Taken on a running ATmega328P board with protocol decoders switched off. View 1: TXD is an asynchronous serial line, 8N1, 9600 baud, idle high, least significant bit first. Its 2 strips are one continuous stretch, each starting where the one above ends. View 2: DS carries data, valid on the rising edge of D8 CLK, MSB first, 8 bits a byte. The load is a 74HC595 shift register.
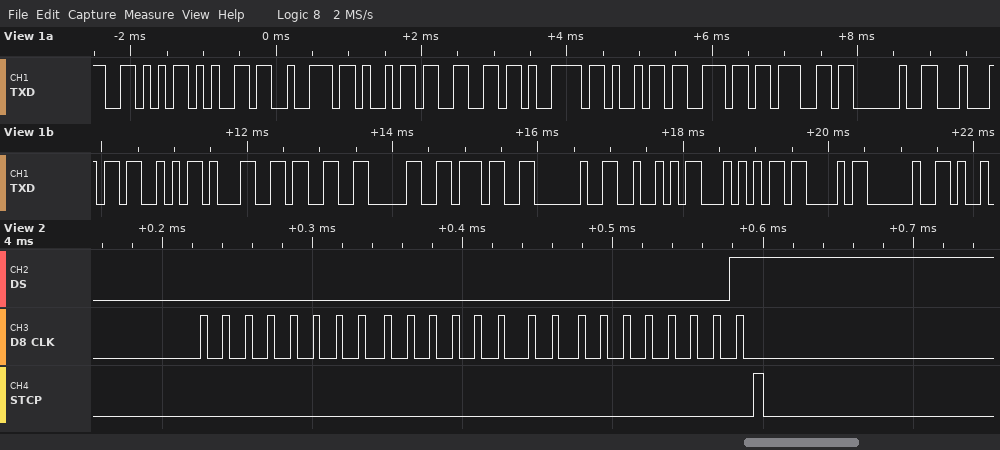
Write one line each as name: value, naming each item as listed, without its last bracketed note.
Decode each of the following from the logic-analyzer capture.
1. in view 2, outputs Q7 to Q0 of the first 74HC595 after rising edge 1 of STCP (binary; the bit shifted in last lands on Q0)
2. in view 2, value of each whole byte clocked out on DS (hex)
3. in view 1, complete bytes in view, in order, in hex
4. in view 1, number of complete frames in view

in view 2, outputs Q7 to Q0 of the first 74HC595 after rising edge 1 of STCP: 00000001
in view 2, value of each whole byte clocked out on DS: 00 00 01
in view 1, complete bytes in view, in order, in hex: 56 65 72 69 66 79 69 6E 67 20 44 53 31 33 30 37 20 52 54 43 20
in view 1, number of complete frames in view: 21
